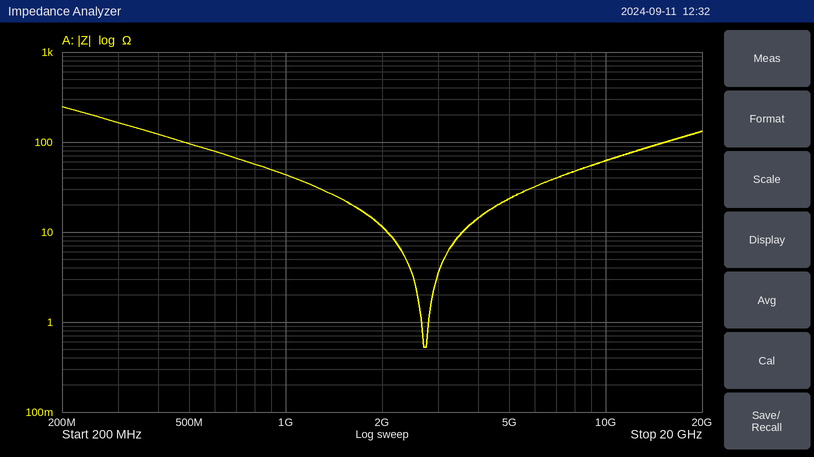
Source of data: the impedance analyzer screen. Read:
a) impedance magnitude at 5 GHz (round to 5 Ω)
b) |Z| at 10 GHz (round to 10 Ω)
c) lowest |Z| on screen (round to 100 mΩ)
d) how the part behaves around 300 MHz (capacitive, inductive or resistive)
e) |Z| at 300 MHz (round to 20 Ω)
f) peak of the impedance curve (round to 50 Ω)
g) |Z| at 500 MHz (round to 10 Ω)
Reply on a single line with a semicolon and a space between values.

25 Ω; 60 Ω; 500 mΩ; capacitive; 160 Ω; 250 Ω; 100 Ω
